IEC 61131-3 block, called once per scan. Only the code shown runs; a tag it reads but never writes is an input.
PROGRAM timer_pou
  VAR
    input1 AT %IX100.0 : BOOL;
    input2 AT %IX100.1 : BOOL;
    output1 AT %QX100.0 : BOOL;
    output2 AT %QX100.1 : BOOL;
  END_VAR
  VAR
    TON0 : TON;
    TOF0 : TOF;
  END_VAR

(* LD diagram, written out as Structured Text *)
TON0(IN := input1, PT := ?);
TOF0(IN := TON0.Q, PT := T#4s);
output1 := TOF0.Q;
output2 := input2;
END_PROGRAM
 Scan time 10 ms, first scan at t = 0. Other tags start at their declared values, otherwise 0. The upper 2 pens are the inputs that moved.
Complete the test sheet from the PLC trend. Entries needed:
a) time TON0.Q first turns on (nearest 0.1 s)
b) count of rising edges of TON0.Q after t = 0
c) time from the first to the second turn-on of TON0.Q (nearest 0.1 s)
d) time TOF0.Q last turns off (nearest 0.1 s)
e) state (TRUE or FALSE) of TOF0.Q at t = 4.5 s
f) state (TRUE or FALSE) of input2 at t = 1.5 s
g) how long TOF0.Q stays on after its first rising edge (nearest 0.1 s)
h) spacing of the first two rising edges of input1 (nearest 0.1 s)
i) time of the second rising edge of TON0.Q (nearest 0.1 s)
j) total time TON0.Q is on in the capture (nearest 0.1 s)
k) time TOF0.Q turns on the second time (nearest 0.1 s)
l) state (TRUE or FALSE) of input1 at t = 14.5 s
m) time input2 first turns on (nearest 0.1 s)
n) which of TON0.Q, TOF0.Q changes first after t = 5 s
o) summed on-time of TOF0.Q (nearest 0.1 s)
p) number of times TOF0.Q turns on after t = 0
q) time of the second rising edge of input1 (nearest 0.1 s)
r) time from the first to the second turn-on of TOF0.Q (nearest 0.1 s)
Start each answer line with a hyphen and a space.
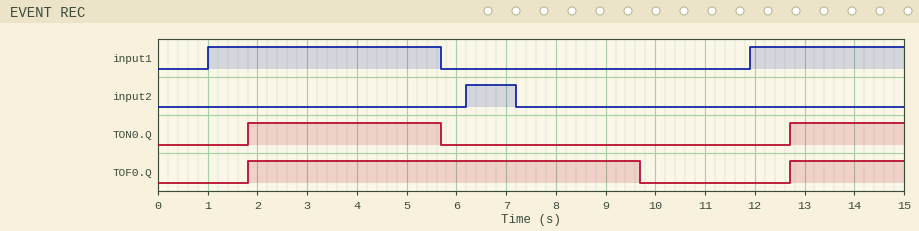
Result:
- 1.8 s
- 2
- 10.9 s
- 9.7 s
- TRUE
- FALSE
- 7.9 s
- 10.9 s
- 12.7 s
- 6.2 s
- 12.7 s
- TRUE
- 6.2 s
- TON0.Q
- 10.2 s
- 2
- 11.9 s
- 10.9 s
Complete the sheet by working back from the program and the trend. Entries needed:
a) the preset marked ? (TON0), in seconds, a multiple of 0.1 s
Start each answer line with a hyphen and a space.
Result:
- 0.8 s
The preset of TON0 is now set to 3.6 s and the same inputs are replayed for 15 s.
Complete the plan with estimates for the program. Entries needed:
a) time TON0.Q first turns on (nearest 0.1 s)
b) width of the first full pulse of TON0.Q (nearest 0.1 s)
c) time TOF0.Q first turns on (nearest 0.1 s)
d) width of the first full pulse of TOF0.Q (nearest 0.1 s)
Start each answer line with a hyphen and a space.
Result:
- 4.6 s
- 1.1 s
- 4.6 s
- 5.1 s
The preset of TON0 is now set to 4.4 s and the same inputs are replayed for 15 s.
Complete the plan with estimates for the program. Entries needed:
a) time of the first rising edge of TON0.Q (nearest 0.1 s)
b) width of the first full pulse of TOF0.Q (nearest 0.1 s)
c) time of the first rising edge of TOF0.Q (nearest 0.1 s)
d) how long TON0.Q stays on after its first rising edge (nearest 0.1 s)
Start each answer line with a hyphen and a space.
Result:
- 5.4 s
- 4.3 s
- 5.4 s
- 0.3 s
